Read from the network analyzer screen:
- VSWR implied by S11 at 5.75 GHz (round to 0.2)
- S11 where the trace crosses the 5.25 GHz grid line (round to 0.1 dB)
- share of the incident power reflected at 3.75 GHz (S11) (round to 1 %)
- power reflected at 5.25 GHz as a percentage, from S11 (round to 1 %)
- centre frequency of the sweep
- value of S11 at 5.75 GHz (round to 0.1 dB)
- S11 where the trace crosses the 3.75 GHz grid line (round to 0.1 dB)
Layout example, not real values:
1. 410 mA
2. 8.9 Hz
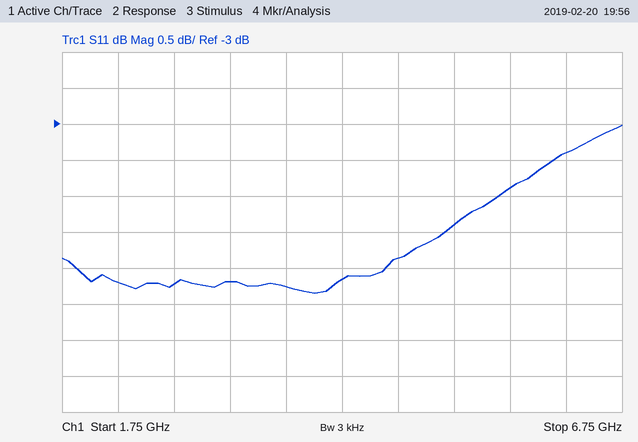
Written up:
1. 4.6
2. -4.4 dB
3. 30 %
4. 36 %
5. 4.25 GHz
6. -3.9 dB
7. -5.3 dB
